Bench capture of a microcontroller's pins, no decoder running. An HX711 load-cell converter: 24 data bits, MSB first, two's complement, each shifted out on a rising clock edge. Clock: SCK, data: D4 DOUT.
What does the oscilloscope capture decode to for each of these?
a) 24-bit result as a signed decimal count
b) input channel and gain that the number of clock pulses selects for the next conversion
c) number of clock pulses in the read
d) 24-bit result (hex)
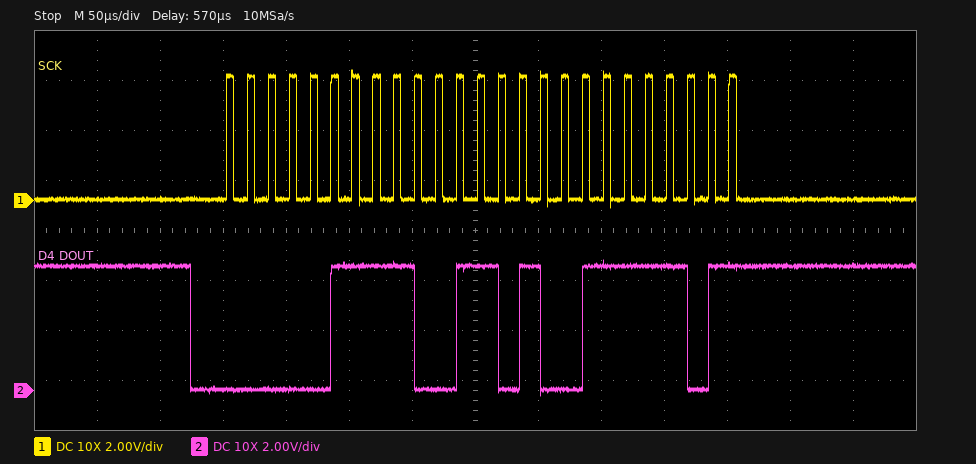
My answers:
498301
channel A, gain 128
25
0x079A7D
